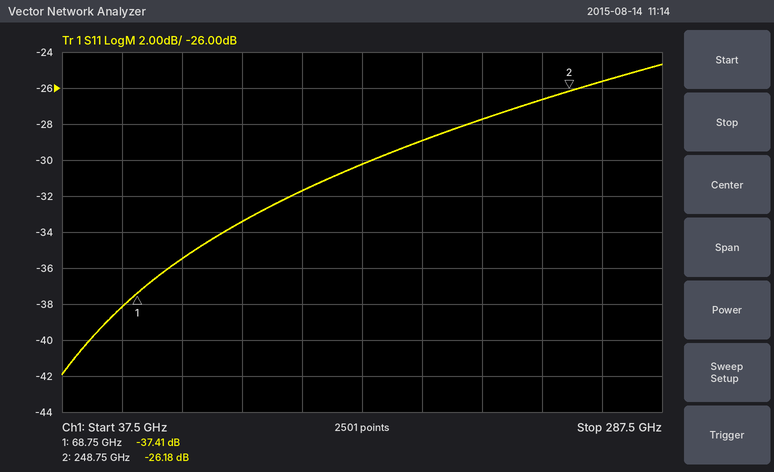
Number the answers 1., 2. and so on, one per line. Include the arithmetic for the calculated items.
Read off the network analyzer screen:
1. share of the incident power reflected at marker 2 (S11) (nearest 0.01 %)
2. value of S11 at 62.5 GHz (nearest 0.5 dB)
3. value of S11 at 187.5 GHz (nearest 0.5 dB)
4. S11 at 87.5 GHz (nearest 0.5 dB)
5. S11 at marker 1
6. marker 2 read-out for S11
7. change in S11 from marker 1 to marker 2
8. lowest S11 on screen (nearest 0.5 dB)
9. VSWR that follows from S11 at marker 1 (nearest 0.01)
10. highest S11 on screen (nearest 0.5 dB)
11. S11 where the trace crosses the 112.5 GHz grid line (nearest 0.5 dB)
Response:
1. 10^(-26.18/10) ≈ 0.24 %
2. -38.0 dB
3. -29.0 dB
4. -35.5 dB
5. -37.41 dB
6. -26.18 dB
7. -26.18 − (-37.41) = 11.23 dB
8. -42.0 dB
9. (1 + 0.0135)/(1 − 0.0135) ≈ 1.03
10. -24.5 dB
11. -33.5 dB
